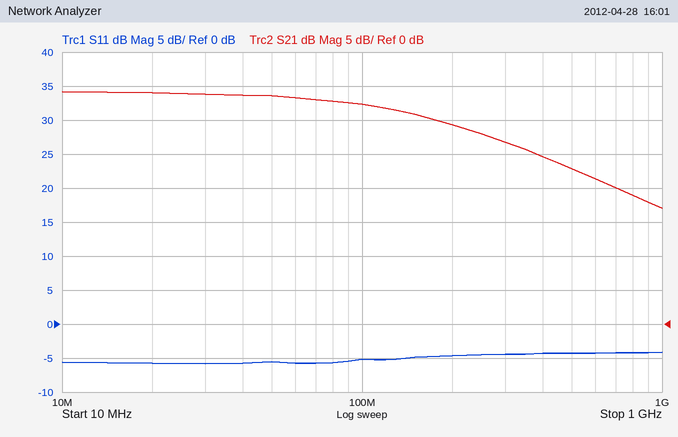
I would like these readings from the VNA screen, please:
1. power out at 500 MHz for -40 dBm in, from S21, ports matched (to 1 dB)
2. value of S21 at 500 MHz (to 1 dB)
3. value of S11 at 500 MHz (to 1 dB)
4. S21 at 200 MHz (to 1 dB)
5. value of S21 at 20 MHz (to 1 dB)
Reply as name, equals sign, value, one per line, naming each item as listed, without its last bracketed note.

power out at 500 MHz for -40 dBm in, from S21, ports matched = -17 dBm
value of S21 at 500 MHz = 23 dB
value of S11 at 500 MHz = -4 dB
S21 at 200 MHz = 29 dB
value of S21 at 20 MHz = 34 dB
